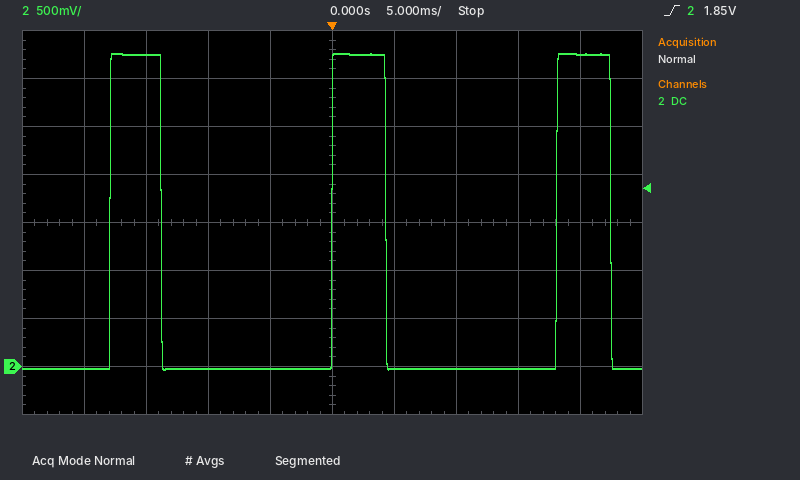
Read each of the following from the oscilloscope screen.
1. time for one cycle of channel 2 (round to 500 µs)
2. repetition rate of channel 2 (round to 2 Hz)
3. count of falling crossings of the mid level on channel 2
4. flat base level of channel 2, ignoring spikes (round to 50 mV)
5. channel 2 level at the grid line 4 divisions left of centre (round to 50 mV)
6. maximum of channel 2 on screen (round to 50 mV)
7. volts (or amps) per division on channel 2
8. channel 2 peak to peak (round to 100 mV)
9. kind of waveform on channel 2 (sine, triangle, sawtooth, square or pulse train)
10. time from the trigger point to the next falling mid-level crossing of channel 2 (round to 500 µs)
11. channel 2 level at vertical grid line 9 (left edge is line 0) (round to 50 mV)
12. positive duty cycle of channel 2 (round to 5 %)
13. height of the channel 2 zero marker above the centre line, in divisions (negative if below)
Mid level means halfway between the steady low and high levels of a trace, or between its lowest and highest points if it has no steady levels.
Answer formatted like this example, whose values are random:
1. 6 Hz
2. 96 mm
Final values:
1. 18.0 ms
2. 56 Hz
3. 3
4. 0 mV
5. 0 mV
6. 3.25 V
7. 500 mV
8. 3.30 V
9. pulse train
10. 4.5 ms
11. 3.25 V
12. 25 %
13. -3.0 div
